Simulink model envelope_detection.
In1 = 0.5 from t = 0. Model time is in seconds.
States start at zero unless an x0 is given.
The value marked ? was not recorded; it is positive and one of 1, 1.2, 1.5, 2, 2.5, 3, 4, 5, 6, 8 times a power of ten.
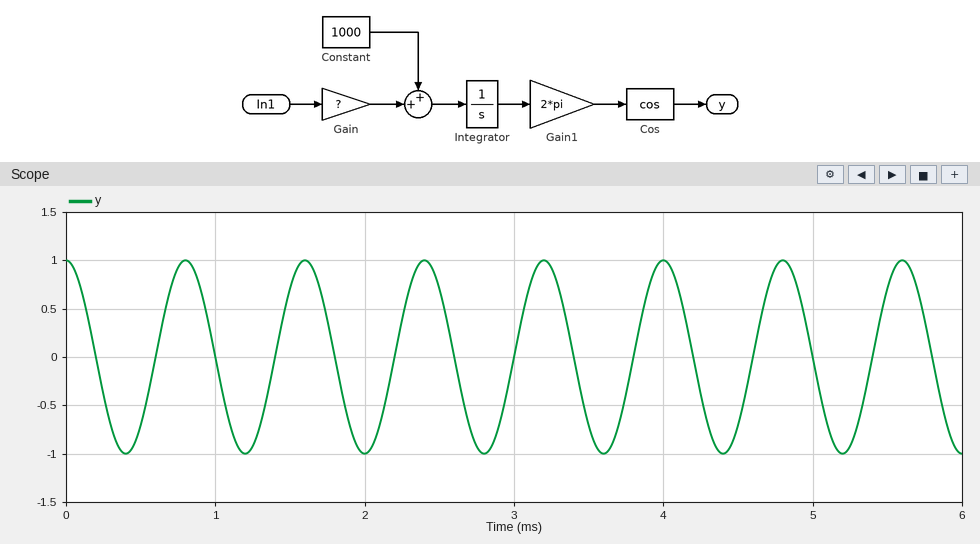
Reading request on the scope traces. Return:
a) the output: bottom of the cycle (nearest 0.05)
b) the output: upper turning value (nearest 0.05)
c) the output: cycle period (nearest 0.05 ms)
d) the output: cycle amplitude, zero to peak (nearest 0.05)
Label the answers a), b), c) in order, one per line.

a) -1.00
b) 1.00
c) 0.80 ms
d) 1.00
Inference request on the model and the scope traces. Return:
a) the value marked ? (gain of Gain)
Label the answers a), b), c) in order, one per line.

a) 500
